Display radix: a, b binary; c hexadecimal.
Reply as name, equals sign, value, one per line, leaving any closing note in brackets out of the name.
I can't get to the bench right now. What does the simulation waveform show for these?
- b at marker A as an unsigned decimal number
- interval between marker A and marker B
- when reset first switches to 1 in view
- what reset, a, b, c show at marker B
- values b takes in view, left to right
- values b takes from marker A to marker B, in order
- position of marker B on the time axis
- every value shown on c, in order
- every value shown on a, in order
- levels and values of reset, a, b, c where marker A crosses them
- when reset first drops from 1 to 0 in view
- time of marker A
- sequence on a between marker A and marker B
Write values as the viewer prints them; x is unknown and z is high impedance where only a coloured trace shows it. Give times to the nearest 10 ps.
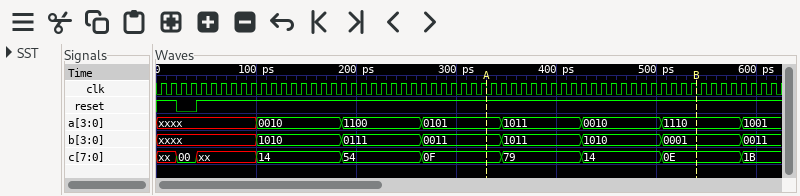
b at marker A as an unsigned decimal number = 3
interval between marker A and marker B = 210 ps
when reset first switches to 1 in view = 40 ps
what reset, a, b, c show at marker B = reset=1, a=1110, b=0001, c=0E
values b takes in view, left to right = xxxx, 1010, 0111, 0011, 1011, 1010, 0001, 0011
values b takes from marker A to marker B, in order = 0011, 1011, 1010, 0001
position of marker B on the time axis = 540 ps
every value shown on c, in order = xx, 00, xx, 14, 54, 0F, 79, 14, 0E, 1B
every value shown on a, in order = xxxx, 0010, 1100, 0101, 1011, 0010, 1110, 1001
levels and values of reset, a, b, c where marker A crosses them = reset=1, a=0101, b=0011, c=0F
when reset first drops from 1 to 0 in view = 20 ps
time of marker A = 330 ps
sequence on a between marker A and marker B = 0101, 1011, 0010, 1110
